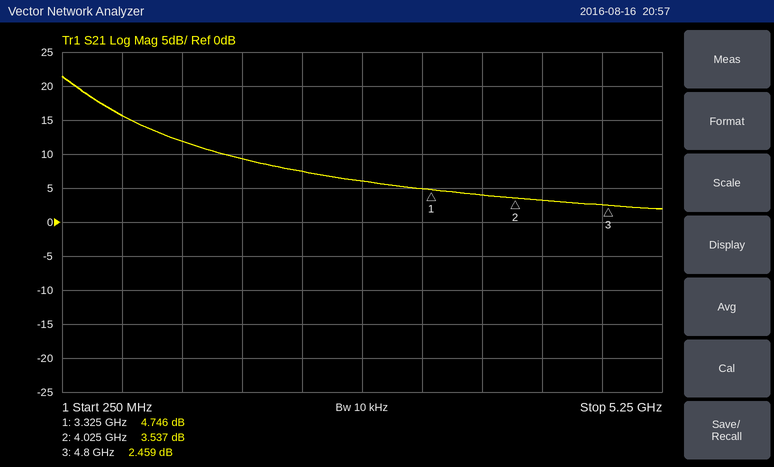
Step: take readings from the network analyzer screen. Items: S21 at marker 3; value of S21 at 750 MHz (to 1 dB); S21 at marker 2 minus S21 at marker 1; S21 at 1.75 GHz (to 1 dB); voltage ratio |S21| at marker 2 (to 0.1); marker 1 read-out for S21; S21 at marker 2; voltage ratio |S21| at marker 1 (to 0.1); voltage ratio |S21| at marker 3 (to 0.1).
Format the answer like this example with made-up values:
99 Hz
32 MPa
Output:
2.459 dB
16 dB
-1.209 dB
9 dB
1.5
4.746 dB
3.537 dB
1.7
1.3
